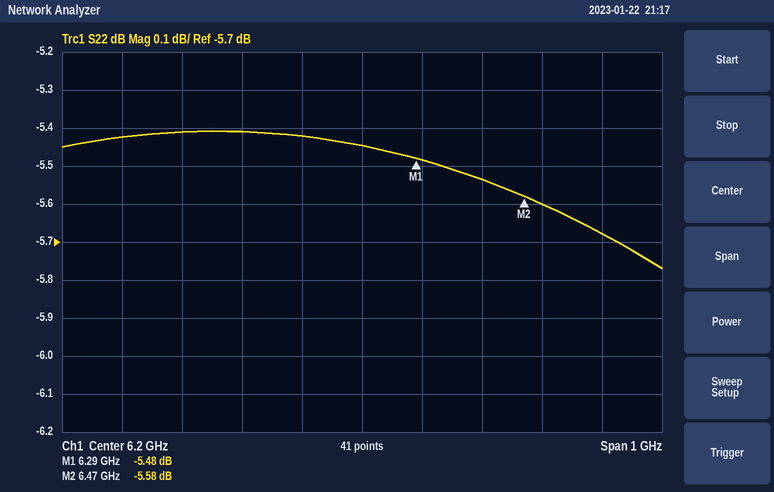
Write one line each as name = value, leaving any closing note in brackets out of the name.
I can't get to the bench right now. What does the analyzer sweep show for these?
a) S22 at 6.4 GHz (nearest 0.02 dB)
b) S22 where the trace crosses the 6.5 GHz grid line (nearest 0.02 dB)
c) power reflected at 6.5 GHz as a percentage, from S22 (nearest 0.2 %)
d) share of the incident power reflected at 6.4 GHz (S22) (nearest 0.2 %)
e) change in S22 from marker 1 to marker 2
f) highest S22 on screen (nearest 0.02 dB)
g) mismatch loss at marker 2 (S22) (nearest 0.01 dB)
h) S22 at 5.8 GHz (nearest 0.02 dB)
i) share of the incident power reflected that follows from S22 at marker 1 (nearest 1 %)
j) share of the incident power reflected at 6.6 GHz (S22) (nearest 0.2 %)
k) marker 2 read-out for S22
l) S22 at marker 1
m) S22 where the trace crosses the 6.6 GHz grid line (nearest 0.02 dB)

S22 at 6.4 GHz = -5.54 dB
S22 where the trace crosses the 6.5 GHz grid line = -5.60 dB
power reflected at 6.5 GHz as a percentage, from S22 = 27.6 %
share of the incident power reflected at 6.4 GHz (S22) = 28.0 %
change in S22 from marker 1 to marker 2 = -0.10 dB
highest S22 on screen = -5.40 dB
mismatch loss at marker 2 (S22) = 1.41 dB
S22 at 5.8 GHz = -5.42 dB
share of the incident power reflected that follows from S22 at marker 1 = 28 %
share of the incident power reflected at 6.6 GHz (S22) = 27.0 %
marker 2 read-out for S22 = -5.58 dB
S22 at marker 1 = -5.48 dB
S22 where the trace crosses the 6.6 GHz grid line = -5.68 dB
